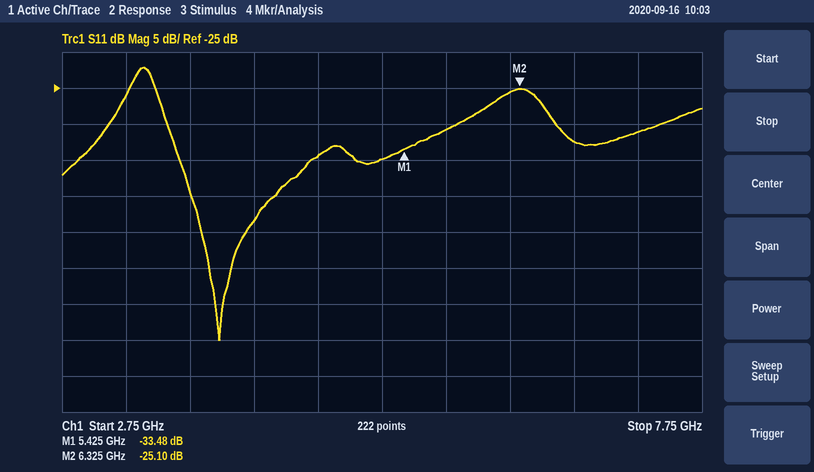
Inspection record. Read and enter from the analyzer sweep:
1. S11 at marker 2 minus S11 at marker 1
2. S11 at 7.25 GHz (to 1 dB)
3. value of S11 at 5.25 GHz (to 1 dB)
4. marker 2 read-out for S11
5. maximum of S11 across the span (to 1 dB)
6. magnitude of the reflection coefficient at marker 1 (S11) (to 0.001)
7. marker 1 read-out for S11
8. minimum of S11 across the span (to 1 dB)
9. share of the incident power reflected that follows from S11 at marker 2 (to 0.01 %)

8.38 dB
-31 dB
-35 dB
-25.10 dB
-22 dB
0.021
-33.48 dB
-60 dB
0.31 %
